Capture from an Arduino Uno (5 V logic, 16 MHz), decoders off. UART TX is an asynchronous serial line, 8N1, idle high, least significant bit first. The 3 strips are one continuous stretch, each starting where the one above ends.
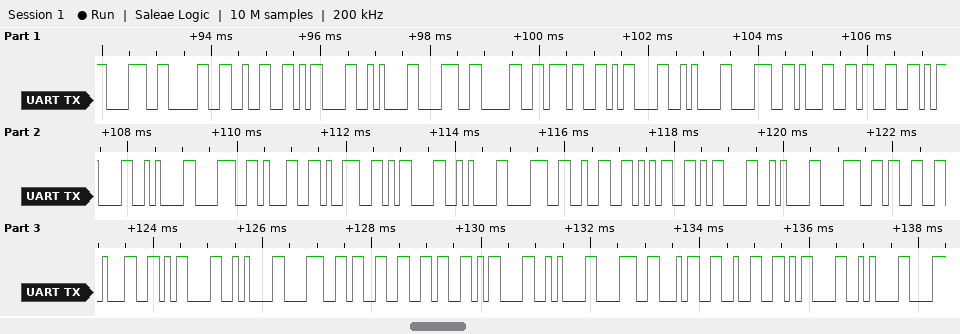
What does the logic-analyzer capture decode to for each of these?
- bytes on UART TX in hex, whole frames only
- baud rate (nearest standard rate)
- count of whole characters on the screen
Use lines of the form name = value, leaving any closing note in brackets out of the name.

bytes on UART TX in hex, whole frames only = 38 30 32 0D 0A 38 30 37 0D 0A 38 31 33 0D 0A 38 31 39 0D 0A 38 32 35 0D 0A 38 33 31 0D 0A 38 33 36 0D 0A 38 34 32 0D 0A
baud rate = 9600 baud
count of whole characters on the screen = 40
